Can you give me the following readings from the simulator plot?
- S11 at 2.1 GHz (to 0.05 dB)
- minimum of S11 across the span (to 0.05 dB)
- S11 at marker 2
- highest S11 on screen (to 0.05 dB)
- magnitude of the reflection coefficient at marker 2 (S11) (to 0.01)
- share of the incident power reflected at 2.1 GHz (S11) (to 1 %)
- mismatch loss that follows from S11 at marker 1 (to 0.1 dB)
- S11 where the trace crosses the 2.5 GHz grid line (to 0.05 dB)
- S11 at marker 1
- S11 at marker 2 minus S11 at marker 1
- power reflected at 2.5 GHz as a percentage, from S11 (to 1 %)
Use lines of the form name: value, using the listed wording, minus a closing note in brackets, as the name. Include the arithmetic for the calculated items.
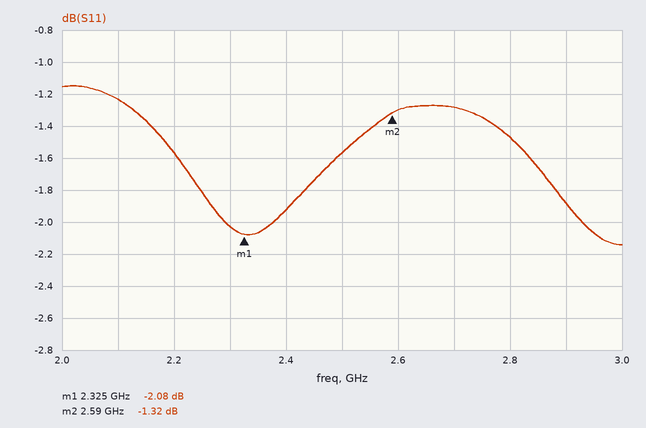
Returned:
S11 at 2.1 GHz: -1.25 dB
minimum of S11 across the span: -2.15 dB
S11 at marker 2: -1.32 dB
highest S11 on screen: -1.15 dB
magnitude of the reflection coefficient at marker 2 (S11): 10^(-1.32/20) ≈ 0.86
share of the incident power reflected at 2.1 GHz (S11): 10^(-1.25/10) ≈ 75 %
mismatch loss that follows from S11 at marker 1: −10 log10(1 − 10^(-2.08/10)) ≈ 4.2 dB
S11 where the trace crosses the 2.5 GHz grid line: -1.55 dB
S11 at marker 1: -2.08 dB
S11 at marker 2 minus S11 at marker 1: -1.32 − (-2.08) = 0.76 dB
power reflected at 2.5 GHz as a percentage, from S11: 10^(-1.55/10) ≈ 70 %
